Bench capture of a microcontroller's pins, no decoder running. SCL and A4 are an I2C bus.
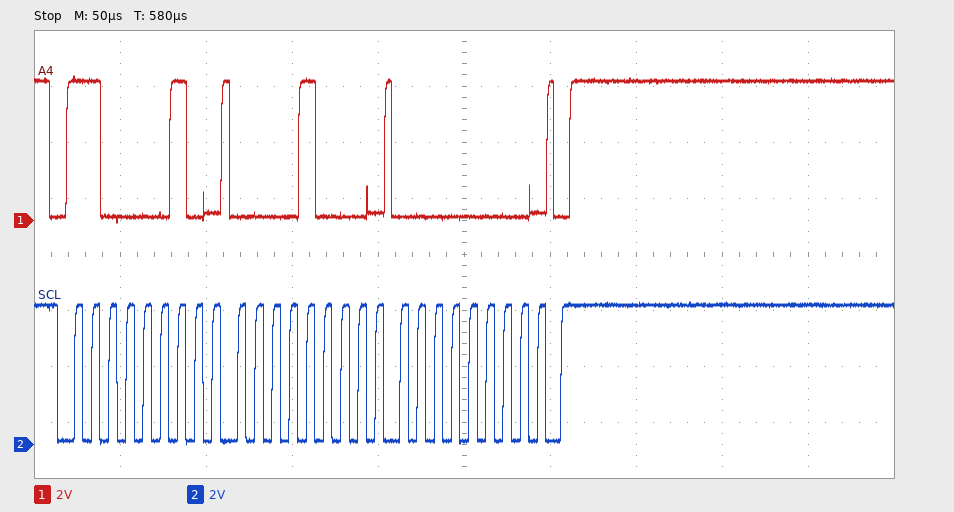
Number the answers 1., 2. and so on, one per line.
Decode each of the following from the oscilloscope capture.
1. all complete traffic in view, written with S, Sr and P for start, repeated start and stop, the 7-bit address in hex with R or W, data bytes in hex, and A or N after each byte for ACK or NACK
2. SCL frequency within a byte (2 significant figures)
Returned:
1. S 61W A 08 A 00 A P
2. 100 kHz
